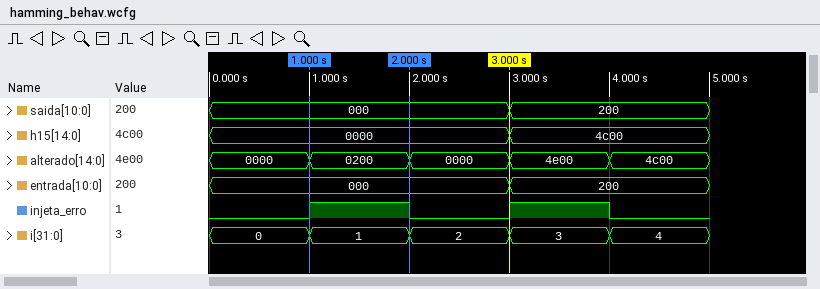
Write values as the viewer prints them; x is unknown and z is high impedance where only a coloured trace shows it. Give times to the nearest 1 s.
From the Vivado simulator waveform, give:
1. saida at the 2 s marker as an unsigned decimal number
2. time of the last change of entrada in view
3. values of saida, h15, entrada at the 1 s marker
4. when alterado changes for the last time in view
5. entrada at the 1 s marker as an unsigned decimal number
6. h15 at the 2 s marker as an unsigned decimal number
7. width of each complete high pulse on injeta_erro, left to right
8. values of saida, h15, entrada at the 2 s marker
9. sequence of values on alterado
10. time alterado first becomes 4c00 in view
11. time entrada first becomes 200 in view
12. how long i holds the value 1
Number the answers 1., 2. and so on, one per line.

1. 0
2. 3 s
3. saida=000, h15=0000, entrada=000
4. 4 s
5. 0
6. 0
7. 1 s, 1 s
8. saida=000, h15=0000, entrada=000
9. 0000, 0200, 0000, 4e00, 4c00
10. 4 s
11. 3 s
12. 1 s
